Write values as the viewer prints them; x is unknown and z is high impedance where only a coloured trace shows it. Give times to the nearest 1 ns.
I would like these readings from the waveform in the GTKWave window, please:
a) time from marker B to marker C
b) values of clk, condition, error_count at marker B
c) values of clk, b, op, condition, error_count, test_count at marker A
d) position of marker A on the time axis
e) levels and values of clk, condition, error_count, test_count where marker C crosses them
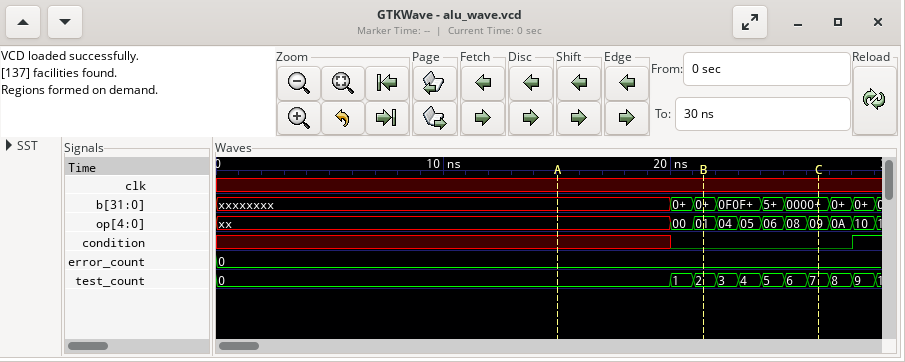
5 ns
clk=x, condition=0, error_count=0
clk=x, b=xxxxxxxx, op=xx, condition=x, error_count=0, test_count=0
15 ns
clk=x, condition=0, error_count=0, test_count=7
